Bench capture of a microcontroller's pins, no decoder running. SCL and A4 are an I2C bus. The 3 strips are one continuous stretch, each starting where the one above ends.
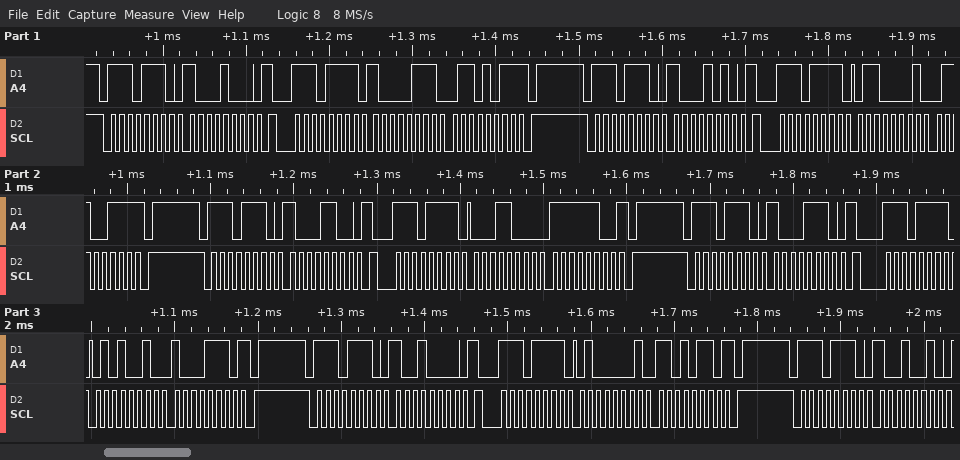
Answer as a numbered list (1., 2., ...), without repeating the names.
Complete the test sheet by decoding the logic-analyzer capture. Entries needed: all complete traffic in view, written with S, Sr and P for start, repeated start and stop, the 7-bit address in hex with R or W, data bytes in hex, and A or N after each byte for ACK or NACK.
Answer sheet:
1. S 77W A 88 A Sr 77R A 87 A 6B N P S 77W A 8A A Sr 77R A 61 A 67 N P S 77W A 8C A Sr 77R A 18 A FC N P S 77W A 8E A Sr 77R A 52 A 8E N P S 77W A 90 A Sr 77R A 41 A D6 N P S 77W A 92 A
